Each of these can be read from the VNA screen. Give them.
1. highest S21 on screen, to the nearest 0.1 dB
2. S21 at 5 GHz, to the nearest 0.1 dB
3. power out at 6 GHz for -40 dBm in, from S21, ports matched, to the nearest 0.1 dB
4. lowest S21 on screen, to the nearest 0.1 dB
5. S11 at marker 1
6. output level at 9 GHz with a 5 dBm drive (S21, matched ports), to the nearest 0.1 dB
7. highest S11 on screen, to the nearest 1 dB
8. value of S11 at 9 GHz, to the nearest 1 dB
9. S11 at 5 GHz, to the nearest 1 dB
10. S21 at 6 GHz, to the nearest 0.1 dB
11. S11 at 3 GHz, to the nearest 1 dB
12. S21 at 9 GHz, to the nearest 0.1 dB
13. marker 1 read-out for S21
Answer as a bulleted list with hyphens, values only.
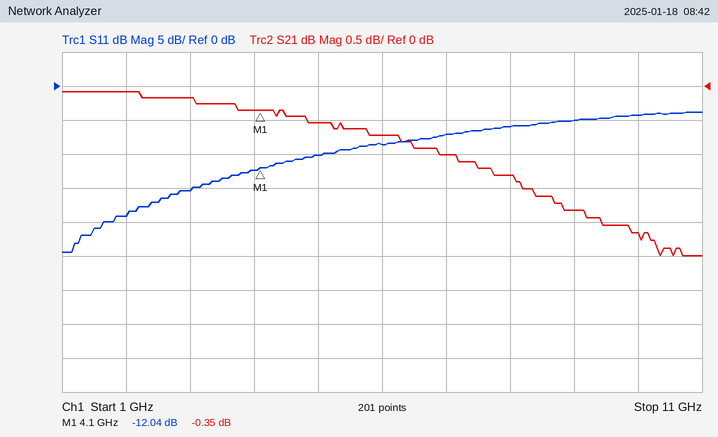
- -0.1 dB
- -0.5 dB
- -40.7 dBm
- -2.5 dB
- -12.04 dB
- 3.2 dBm
- -4 dB
- -5 dB
- -10 dB
- -0.7 dB
- -15 dB
- -1.8 dB
- -0.35 dB
